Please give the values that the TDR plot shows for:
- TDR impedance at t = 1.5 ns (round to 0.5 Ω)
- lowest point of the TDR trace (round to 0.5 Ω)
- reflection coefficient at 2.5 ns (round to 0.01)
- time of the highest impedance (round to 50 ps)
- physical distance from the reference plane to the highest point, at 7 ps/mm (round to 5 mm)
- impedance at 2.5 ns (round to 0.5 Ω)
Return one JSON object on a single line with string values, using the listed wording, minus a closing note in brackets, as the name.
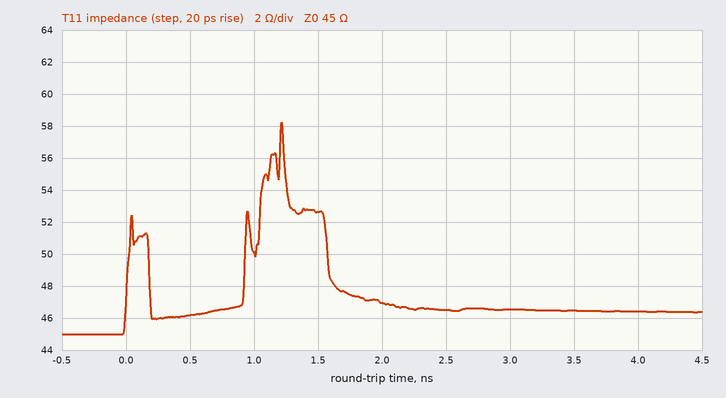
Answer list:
{"TDR impedance at t = 1.5 ns": "52.5 Ω", "lowest point of the TDR trace": "45.0 Ω", "reflection coefficient at 2.5 ns": "+0.02", "time of the highest impedance": "1.20 ns", "physical distance from the reference plane to the highest point, at 7 ps/mm": "85 mm", "impedance at 2.5 ns": "46.5 Ω"}
